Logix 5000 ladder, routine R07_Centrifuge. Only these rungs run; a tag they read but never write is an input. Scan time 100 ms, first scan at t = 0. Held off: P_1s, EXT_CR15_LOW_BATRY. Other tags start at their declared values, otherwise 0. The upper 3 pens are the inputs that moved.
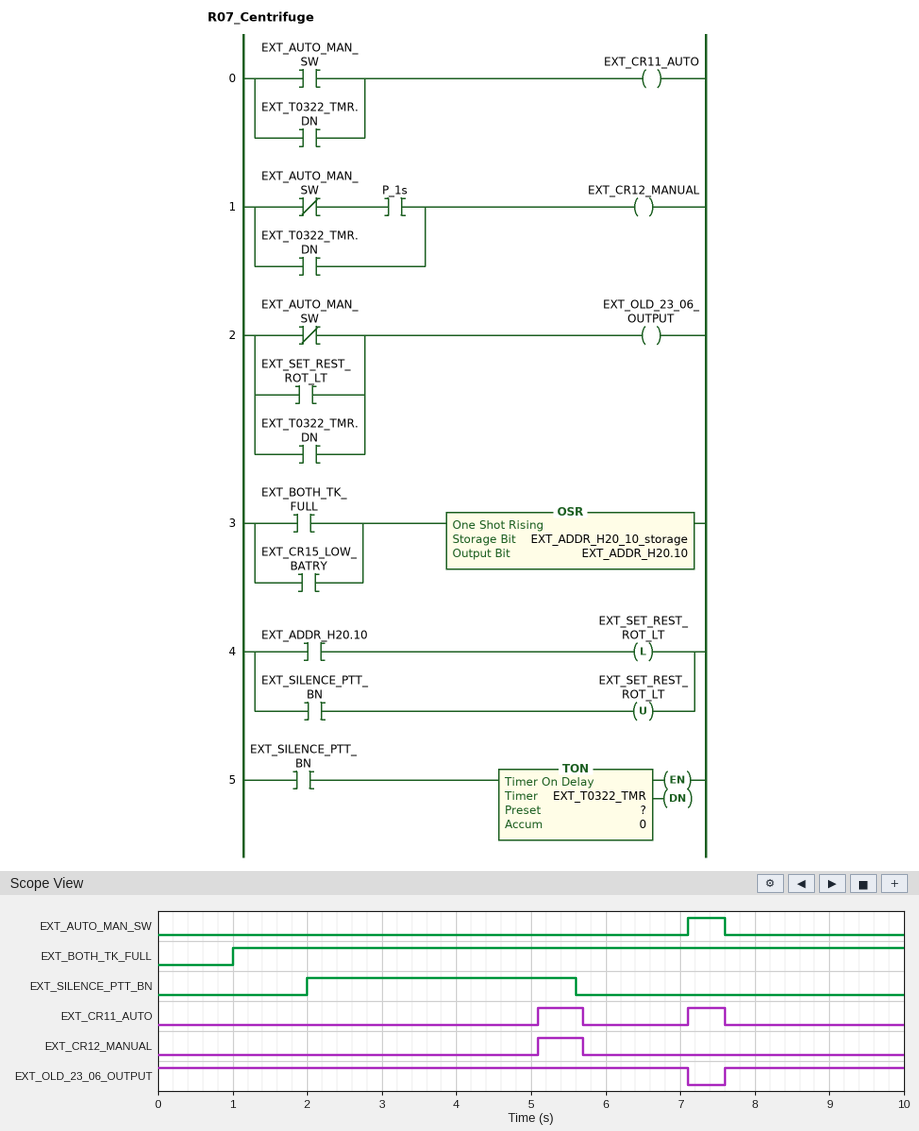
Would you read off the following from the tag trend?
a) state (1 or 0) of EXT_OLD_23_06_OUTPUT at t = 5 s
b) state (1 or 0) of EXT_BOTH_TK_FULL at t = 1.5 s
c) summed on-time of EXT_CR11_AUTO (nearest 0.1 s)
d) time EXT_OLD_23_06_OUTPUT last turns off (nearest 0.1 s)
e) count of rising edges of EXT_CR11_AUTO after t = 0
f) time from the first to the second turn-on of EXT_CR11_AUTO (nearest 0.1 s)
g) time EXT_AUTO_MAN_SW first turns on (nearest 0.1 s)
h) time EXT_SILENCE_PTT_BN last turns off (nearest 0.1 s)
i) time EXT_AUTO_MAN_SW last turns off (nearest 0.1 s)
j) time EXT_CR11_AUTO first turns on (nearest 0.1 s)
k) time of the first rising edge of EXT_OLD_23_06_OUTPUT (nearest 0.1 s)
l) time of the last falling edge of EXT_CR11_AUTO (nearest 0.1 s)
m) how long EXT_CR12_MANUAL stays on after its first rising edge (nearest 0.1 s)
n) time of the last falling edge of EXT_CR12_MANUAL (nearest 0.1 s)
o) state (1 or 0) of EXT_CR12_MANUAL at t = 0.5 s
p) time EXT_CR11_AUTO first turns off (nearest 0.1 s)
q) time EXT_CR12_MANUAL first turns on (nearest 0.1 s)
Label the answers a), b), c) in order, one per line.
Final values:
a) 1
b) 1
c) 1.1 s
d) 7.1 s
e) 2
f) 2.0 s
g) 7.1 s
h) 5.6 s
i) 7.6 s
j) 5.1 s
k) 7.6 s
l) 7.6 s
m) 0.6 s
n) 5.7 s
o) 0
p) 5.7 s
q) 5.1 s
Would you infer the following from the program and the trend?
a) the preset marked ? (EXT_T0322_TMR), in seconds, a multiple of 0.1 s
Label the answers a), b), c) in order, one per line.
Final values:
a) 3.0 s
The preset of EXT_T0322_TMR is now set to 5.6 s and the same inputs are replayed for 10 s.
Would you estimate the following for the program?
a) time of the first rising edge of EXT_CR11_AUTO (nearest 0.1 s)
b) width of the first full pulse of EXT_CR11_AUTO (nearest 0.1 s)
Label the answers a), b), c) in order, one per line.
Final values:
a) 7.1 s
b) 0.5 s
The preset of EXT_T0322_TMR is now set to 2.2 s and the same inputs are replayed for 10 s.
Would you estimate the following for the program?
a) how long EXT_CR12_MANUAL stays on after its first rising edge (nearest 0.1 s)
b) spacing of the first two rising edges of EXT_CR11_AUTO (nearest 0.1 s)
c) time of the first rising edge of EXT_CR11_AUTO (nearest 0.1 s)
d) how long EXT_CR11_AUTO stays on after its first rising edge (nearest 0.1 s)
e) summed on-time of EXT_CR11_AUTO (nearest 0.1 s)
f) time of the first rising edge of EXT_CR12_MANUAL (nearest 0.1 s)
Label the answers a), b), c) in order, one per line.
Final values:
a) 1.4 s
b) 2.8 s
c) 4.3 s
d) 1.4 s
e) 1.9 s
f) 4.3 s
